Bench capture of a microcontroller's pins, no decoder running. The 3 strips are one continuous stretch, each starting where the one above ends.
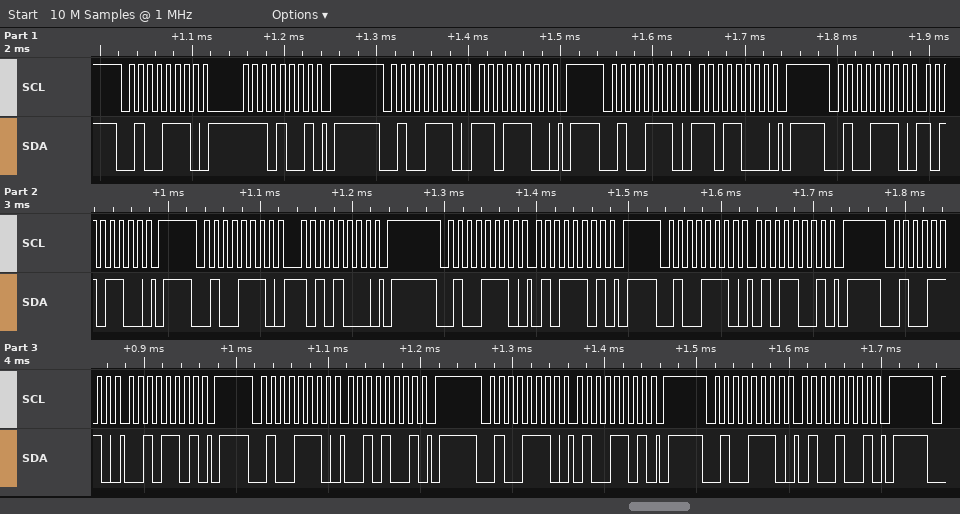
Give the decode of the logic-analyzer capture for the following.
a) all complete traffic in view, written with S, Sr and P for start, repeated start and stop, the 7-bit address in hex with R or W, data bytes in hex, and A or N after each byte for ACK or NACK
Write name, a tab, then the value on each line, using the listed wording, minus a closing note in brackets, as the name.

all complete traffic in view, written with S, Sr and P for start, repeated start and stop, the 7-bit address in hex with R or W, data bytes in hex, and A or N after each byte for ACK or NACK	S 27W A E9 A P S 27W A DC A P S 27W A D8 A P S 27W A AC A P S 27W A A8 A P S 27W A 5D A P S 27W A 59 A P S 27W A 2D A P S 27W A 29 A P S 27W A 4D A P S 27W A 49 A P
